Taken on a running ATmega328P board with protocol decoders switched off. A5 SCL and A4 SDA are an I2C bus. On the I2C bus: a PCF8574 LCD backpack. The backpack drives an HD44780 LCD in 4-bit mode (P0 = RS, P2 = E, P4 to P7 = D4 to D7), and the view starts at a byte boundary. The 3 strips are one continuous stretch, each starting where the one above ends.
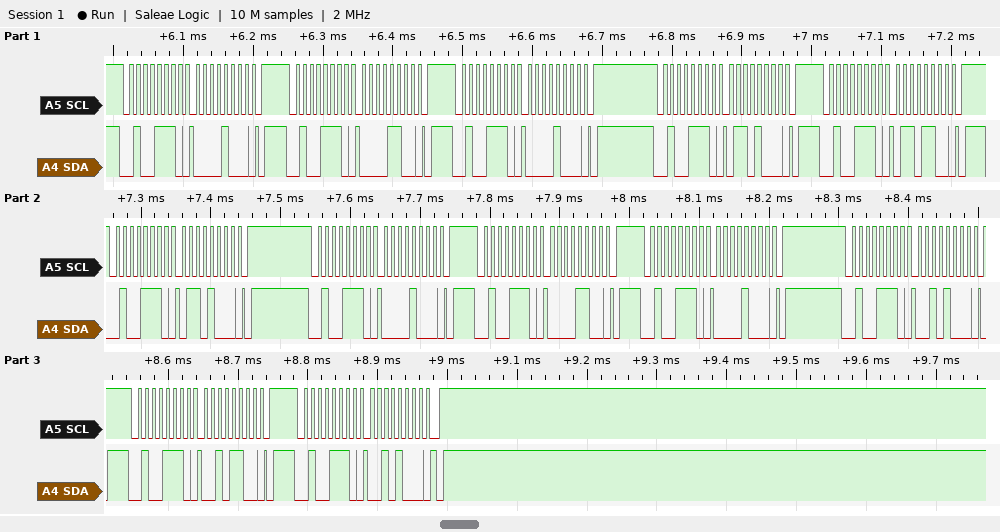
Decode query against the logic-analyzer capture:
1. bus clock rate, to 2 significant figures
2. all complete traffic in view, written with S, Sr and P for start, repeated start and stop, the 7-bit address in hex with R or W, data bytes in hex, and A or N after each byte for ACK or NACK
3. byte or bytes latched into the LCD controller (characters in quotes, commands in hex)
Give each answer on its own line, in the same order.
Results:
100 kHz
S 27W A 08 A P S 27W A 0C A P S 27W A 08 A P S 27W A 68 A P S 27W A 6C A P S 27W A 68 A P S 27W A 08 A P S 27W A 0C A P S 27W A 08 A P S 27W A 28 A P S 27W A 2C A P S 27W A 28 A P
0x06 0x02
